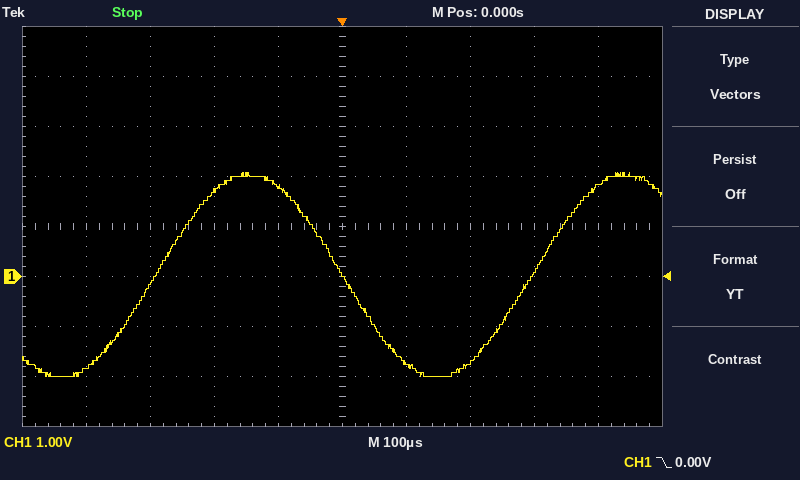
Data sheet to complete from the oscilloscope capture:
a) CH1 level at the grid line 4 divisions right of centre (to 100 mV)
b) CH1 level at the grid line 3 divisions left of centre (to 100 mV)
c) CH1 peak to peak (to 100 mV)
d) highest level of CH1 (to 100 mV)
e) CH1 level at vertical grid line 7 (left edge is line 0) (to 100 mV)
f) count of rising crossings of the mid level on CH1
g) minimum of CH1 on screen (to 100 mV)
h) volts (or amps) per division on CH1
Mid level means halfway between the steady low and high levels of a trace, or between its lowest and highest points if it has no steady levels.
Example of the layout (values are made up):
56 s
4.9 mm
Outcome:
1.8 V
-200 mV
4.1 V
2.1 V
-1.7 V
2
-2.0 V
1 V
